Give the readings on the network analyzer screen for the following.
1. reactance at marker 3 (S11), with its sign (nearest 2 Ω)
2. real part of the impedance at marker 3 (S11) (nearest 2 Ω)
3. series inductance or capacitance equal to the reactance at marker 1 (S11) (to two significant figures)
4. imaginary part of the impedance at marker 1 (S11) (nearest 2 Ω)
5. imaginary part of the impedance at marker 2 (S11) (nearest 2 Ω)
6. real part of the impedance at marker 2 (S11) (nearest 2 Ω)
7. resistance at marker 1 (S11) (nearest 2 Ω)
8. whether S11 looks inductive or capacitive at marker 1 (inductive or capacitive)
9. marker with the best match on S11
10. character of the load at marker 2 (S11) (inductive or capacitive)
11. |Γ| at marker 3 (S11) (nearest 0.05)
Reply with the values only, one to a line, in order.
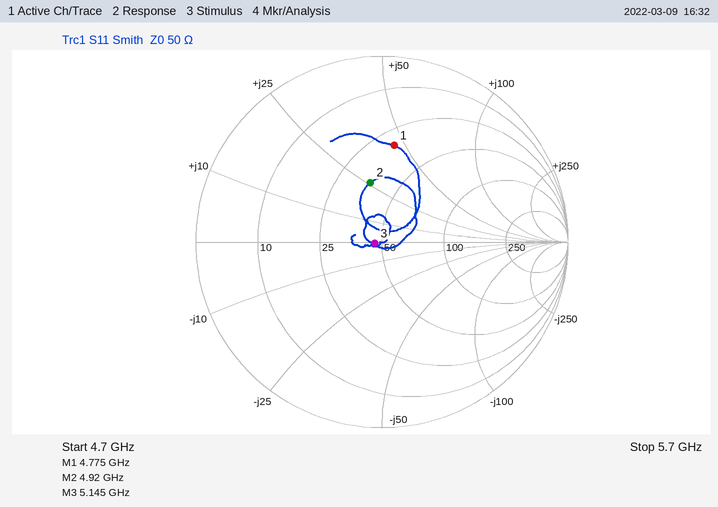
0 Ω
46 Ω
1.5 nH
+46 Ω
+26 Ω
36 Ω
32 Ω
inductive
marker 3
inductive
0.05
